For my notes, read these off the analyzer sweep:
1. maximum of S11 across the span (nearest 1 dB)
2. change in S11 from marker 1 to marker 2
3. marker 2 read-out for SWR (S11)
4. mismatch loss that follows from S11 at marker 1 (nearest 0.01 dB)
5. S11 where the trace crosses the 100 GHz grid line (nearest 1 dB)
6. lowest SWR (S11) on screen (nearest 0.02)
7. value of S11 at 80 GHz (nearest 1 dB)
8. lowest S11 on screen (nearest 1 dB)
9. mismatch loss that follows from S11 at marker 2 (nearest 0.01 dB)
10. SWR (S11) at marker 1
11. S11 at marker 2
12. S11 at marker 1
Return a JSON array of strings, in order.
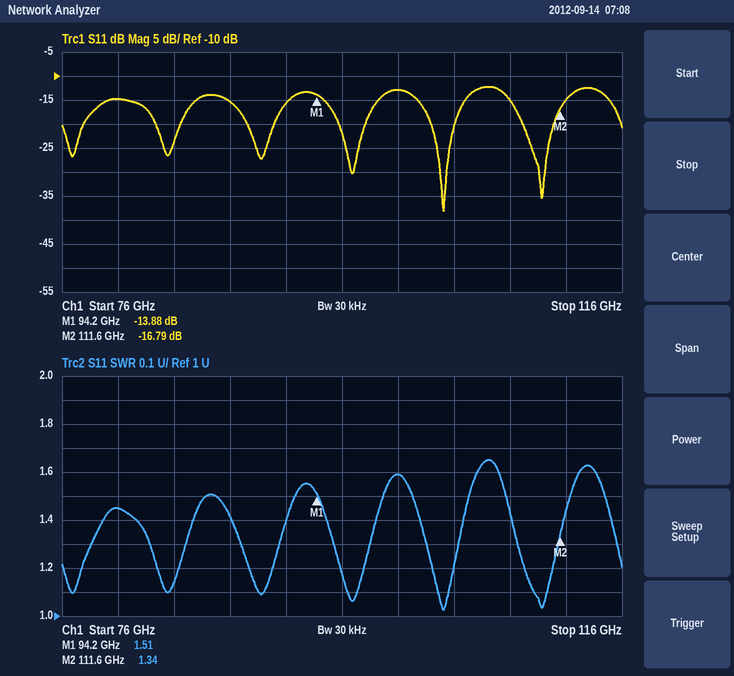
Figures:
["-12 dB", "-2.91 dB", "1.34", "0.18 dB", "-13 dB", "1.02", "-15 dB", "-38 dB", "0.09 dB", "1.51", "-16.79 dB", "-13.88 dB"]
